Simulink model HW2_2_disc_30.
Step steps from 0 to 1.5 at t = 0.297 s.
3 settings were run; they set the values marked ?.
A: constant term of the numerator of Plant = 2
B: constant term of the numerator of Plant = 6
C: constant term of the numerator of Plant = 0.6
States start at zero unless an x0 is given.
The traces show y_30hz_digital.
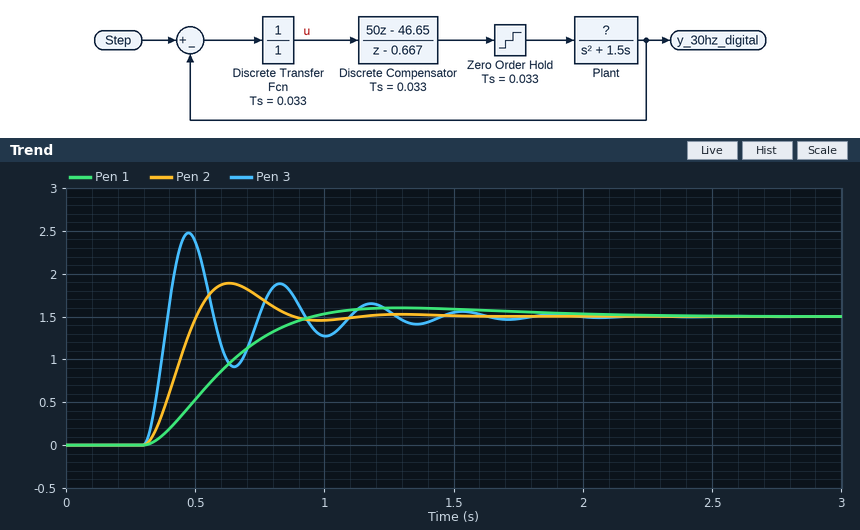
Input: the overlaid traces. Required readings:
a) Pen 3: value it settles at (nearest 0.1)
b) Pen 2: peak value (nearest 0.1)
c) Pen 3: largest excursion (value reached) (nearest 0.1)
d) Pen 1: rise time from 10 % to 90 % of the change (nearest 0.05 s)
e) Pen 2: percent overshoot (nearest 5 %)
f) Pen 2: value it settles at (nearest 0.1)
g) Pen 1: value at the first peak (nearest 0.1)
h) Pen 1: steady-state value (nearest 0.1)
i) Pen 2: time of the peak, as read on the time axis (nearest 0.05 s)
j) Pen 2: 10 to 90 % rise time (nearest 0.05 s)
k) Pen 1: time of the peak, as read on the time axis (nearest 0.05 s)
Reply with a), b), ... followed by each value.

a) 1.5
b) 1.9
c) 2.5
d) 0.45 s
e) 25 %
f) 1.5
g) 1.6
h) 1.5
i) 0.65 s
j) 0.15 s
k) 1.30 s
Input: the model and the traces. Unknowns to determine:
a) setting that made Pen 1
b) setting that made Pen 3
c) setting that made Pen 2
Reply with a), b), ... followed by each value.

a) C
b) B
c) A
